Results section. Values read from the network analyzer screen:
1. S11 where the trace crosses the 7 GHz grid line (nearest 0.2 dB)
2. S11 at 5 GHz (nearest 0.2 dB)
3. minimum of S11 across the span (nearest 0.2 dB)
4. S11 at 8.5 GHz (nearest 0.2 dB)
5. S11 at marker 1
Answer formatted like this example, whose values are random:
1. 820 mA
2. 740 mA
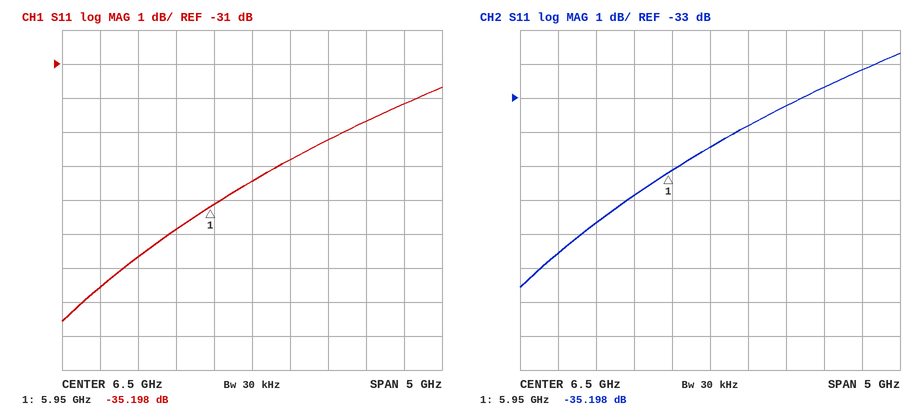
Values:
1. -33.8 dB
2. -36.6 dB
3. -38.6 dB
4. -32.2 dB
5. -35.198 dB
